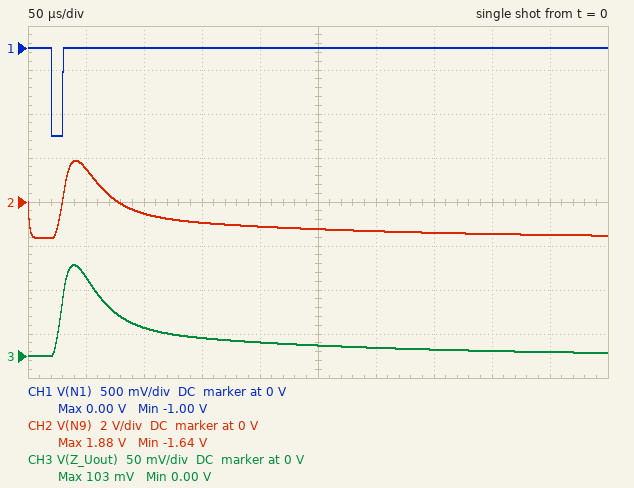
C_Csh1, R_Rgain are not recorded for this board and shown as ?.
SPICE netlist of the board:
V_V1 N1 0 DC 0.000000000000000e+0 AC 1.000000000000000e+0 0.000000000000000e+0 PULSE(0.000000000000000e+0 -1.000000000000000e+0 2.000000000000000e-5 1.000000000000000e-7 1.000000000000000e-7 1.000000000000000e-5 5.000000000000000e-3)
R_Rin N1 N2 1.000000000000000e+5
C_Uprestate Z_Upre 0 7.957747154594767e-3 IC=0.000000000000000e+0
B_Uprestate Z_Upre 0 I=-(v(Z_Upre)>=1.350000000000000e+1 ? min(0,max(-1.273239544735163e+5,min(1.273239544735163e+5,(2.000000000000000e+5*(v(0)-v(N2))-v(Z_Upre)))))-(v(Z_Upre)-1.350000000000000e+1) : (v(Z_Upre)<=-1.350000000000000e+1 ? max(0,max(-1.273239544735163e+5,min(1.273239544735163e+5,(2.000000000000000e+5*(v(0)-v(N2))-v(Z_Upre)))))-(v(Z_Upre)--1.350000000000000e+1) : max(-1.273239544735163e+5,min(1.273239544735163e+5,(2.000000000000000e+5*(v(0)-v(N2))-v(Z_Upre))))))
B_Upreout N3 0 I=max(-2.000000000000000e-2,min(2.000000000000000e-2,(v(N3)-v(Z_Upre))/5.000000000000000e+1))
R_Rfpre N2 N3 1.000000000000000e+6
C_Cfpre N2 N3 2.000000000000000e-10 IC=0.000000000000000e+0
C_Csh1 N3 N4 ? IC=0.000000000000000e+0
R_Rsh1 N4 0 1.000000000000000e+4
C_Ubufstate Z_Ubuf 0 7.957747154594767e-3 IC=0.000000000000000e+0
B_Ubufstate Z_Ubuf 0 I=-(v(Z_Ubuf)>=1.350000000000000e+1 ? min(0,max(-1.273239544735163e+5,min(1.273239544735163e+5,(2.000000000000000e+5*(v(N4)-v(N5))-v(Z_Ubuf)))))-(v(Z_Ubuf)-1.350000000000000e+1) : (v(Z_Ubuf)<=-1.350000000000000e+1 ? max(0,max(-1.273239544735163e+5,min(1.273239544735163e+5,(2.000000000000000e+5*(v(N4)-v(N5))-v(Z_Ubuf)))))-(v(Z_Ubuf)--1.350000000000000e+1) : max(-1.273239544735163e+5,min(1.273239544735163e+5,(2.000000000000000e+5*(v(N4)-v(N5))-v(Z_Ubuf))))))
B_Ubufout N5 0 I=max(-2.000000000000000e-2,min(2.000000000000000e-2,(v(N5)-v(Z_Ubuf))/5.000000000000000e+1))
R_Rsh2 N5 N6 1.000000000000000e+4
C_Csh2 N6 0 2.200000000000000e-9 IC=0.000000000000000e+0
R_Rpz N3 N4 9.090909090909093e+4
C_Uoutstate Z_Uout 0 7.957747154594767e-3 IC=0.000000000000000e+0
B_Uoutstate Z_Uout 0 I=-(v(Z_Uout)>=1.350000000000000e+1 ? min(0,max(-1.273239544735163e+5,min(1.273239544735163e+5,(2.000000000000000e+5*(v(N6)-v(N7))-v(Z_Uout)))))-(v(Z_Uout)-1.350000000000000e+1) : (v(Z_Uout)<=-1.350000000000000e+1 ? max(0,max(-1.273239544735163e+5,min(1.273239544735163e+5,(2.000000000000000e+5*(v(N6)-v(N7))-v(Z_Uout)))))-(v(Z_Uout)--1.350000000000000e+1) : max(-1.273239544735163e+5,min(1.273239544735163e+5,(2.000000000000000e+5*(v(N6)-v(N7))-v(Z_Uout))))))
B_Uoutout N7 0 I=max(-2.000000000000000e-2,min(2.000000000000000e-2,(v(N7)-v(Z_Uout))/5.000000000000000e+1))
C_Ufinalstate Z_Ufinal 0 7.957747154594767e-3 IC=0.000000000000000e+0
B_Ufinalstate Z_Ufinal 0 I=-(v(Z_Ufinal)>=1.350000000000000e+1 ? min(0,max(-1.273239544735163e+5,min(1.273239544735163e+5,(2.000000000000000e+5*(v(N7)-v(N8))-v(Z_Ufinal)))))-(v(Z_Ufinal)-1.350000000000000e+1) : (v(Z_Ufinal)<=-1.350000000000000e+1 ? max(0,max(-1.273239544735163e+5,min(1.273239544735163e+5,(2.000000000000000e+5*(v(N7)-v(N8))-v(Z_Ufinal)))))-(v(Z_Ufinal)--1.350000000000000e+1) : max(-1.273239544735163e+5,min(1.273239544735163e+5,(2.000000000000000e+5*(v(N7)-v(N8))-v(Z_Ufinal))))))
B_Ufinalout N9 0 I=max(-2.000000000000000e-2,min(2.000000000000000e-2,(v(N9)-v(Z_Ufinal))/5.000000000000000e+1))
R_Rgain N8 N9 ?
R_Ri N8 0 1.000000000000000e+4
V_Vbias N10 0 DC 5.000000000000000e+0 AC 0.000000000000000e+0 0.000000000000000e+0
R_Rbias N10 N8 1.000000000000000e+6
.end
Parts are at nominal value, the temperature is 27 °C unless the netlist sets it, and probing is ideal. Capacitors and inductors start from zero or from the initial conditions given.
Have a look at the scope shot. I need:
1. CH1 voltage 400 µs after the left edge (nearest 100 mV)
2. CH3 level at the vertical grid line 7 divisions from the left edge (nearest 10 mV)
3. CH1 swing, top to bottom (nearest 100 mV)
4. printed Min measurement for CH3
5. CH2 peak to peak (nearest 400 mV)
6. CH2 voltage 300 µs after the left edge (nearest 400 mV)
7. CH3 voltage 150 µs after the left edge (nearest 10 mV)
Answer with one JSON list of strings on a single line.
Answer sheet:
["0 V", "10 mV", "1.0 V", "0.00 V", "3.6 V", "-1.2 V", "20 mV"]
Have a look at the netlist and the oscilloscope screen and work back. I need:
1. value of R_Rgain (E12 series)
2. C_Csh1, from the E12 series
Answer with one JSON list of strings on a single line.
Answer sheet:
["330 kΩ", "820 pF"]
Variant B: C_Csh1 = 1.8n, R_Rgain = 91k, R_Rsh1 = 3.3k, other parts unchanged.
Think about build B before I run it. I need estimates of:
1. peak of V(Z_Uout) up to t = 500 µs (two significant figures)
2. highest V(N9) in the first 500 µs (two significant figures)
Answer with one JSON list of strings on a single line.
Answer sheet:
["80 mV", "360 mV"]
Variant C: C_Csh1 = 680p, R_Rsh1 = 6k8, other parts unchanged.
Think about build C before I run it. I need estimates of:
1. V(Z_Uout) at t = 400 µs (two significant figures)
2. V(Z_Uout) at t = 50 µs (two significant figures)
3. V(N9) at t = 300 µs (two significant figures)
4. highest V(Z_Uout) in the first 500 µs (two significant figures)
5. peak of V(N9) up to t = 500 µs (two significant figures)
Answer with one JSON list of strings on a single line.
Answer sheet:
["4.3 mV", "53 mV", "-1.4 V", "69 mV", "710 mV"]
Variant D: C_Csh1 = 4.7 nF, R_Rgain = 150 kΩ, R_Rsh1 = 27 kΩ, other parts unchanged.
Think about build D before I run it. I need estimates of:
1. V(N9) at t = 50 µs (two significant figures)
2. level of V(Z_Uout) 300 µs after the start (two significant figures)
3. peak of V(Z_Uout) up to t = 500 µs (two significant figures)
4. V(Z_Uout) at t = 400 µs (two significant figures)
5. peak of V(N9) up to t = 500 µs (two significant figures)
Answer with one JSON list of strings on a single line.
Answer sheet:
["3.7 V", "-14 mV", "300 mV", "-23 mV", "4.1 V"]
